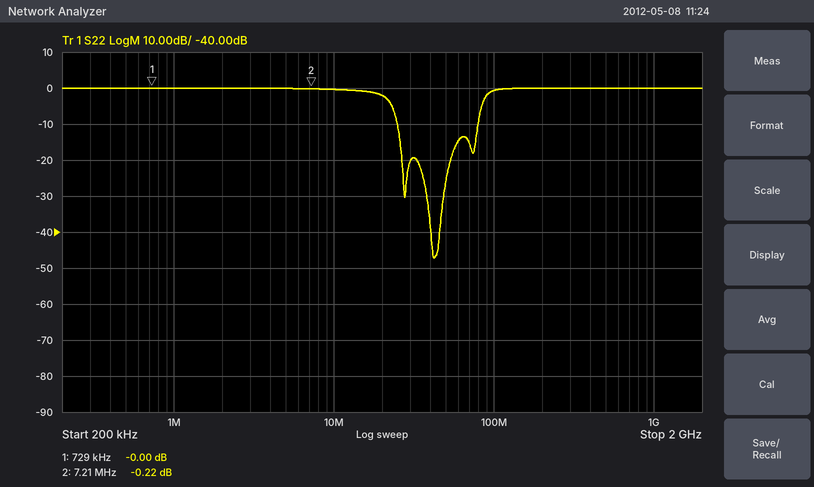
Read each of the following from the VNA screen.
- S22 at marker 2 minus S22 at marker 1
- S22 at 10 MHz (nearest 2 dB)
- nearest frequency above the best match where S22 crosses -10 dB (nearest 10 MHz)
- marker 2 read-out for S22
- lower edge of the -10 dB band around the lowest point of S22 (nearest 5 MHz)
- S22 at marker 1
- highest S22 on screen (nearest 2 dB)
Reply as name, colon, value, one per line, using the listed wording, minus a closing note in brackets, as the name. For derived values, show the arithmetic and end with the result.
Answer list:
S22 at marker 2 minus S22 at marker 1: -0.22 − (-0) = -0.22 dB
S22 at 10 MHz: 0 dB
nearest frequency above the best match where S22 crosses -10 dB: 80 MHz
marker 2 read-out for S22: -0.22 dB
lower edge of the -10 dB band around the lowest point of S22: 25 MHz
S22 at marker 1: -0.00 dB
highest S22 on screen: 0 dB
